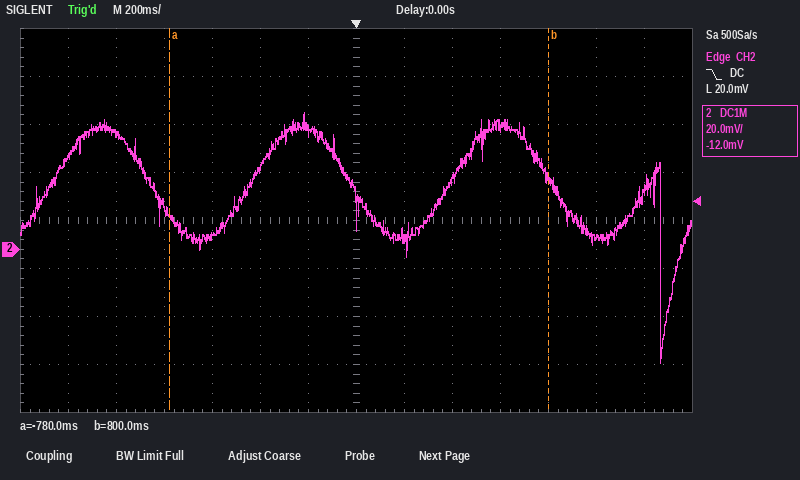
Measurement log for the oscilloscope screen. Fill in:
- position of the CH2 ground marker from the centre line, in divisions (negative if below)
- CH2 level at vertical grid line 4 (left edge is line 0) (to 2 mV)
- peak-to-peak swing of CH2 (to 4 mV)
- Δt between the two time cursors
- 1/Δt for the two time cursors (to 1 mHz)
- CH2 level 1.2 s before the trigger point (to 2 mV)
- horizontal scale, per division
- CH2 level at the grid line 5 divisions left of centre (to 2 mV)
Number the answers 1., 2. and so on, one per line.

1. -0.6 div
2. 6 mV
3. 104 mV
4. 1.58 s
5. 633 mHz
6. 38 mV
7. 200 ms
8. 48 mV
